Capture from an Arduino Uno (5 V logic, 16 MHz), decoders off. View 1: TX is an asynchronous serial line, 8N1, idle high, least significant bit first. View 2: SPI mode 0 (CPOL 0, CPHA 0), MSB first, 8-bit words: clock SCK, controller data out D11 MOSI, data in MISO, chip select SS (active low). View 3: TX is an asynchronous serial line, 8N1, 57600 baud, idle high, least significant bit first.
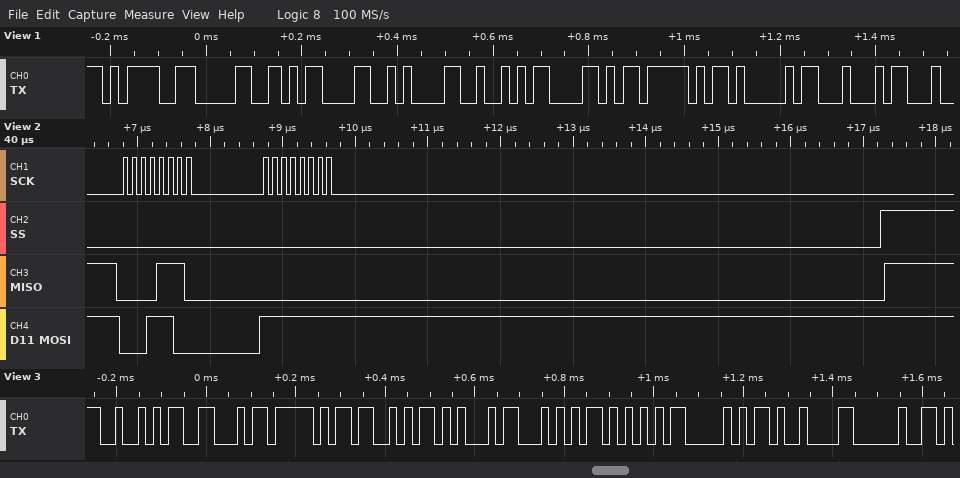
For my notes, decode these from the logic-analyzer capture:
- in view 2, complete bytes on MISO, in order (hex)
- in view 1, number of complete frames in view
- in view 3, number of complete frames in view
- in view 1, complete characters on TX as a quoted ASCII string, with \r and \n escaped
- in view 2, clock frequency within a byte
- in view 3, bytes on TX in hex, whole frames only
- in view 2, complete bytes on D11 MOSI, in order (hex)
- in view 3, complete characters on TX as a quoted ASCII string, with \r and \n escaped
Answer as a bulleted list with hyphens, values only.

- 0E 00
- 9
- 10
- "=0\r\nRX_AD"
- 8 MHz
- 52 46 5F 53 45 54 55 50 09 20
- 1C FF
- "RF_SETUP\t "
